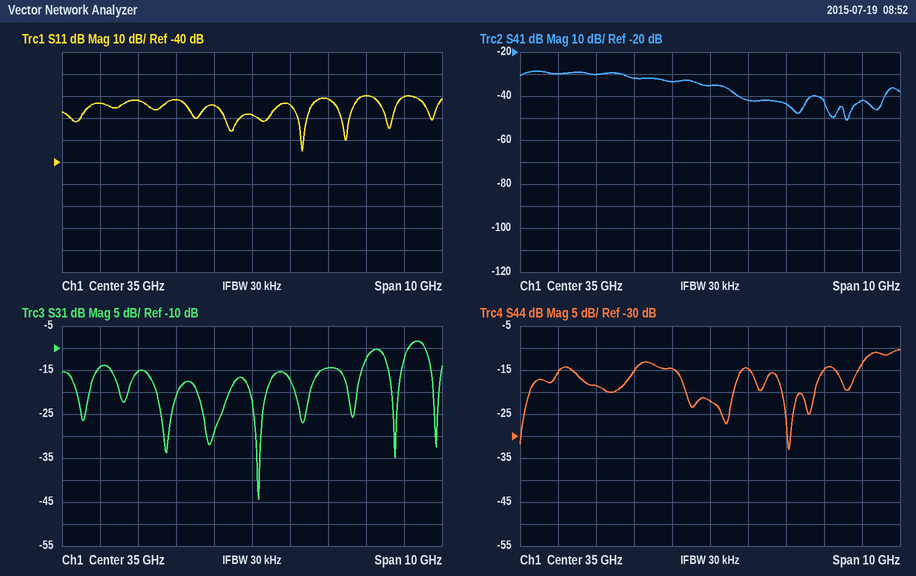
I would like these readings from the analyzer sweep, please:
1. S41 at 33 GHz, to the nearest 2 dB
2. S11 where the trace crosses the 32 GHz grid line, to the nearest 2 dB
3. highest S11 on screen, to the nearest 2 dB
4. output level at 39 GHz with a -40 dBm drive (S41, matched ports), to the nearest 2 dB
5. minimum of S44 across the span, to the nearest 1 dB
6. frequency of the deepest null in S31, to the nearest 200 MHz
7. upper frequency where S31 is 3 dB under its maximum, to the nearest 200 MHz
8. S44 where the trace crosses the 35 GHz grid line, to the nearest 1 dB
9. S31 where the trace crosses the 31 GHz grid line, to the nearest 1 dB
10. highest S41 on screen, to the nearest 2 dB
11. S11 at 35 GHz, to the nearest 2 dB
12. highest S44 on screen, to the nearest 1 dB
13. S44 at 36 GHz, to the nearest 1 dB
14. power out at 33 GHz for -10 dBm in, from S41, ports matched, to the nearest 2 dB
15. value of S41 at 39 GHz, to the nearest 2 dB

-32 dB
-12 dB
-10 dB
-82 dBm
-33 dB
35.2 GHz
39.6 GHz
-22 dB
-14 dB
-28 dB
-18 dB
-10 dB
-15 dB
-42 dBm
-42 dB
